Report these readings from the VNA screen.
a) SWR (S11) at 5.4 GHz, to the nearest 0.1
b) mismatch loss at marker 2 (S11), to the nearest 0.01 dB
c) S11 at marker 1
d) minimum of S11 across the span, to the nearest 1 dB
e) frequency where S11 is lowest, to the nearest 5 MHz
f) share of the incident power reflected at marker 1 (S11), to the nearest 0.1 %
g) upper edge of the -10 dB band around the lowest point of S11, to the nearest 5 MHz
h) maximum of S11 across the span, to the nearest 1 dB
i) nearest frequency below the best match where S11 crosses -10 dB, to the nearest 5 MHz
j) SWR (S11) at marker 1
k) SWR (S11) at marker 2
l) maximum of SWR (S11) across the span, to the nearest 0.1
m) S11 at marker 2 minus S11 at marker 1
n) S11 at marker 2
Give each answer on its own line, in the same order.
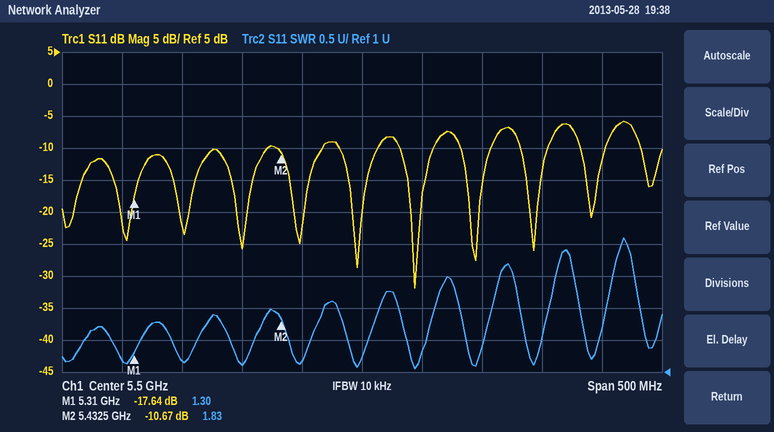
1.1
0.39 dB
-17.64 dB
-32 dB
5.545 GHz
1.7 %
5.560 GHz
-6 dB
5.530 GHz
1.30
1.83
3.1
6.97 dB
-10.67 dB
